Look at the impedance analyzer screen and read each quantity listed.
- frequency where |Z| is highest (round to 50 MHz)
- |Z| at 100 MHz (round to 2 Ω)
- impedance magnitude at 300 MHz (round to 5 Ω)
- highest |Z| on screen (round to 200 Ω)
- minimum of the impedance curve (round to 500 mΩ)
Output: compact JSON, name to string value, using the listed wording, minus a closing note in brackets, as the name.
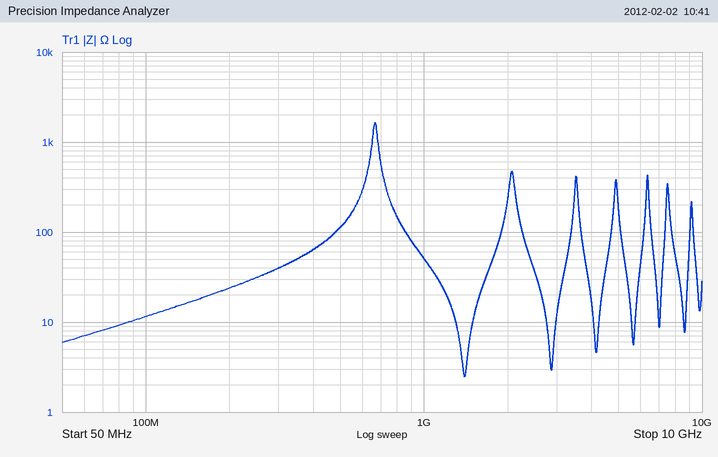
{"frequency where |Z| is highest": "650 MHz", "|Z| at 100 MHz": "12 Ω", "impedance magnitude at 300 MHz": "40 Ω", "highest |Z| on screen": "1.6 kΩ", "minimum of the impedance curve": "2.5 Ω"}
